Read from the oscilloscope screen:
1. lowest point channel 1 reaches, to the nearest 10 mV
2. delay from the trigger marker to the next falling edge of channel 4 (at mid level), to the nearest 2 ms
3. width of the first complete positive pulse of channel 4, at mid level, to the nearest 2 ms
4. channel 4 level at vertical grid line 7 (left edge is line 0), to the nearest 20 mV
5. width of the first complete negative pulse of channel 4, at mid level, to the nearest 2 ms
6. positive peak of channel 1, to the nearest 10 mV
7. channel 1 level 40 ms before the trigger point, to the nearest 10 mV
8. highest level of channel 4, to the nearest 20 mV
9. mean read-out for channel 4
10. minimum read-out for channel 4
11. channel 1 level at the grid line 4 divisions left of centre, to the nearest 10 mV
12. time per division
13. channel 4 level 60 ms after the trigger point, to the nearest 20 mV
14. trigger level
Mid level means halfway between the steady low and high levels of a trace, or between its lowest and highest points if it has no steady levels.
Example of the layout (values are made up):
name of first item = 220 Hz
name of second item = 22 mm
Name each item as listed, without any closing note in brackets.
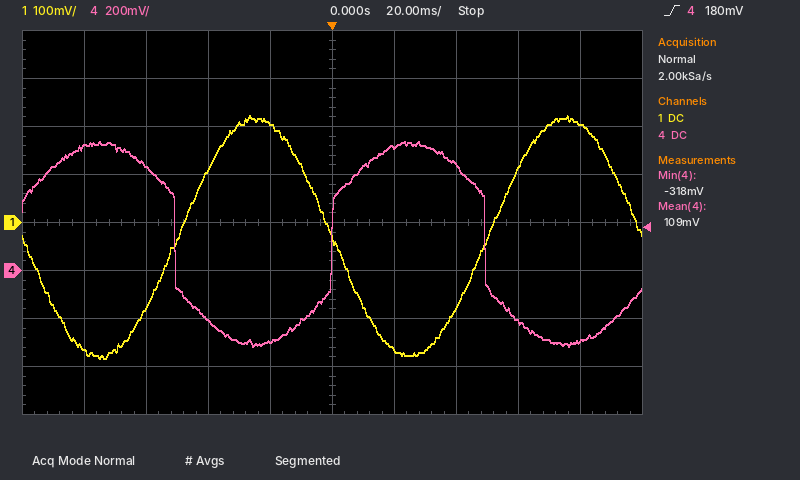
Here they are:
lowest point channel 1 reaches, to the nearest 10 mV = -280 mV
delay from the trigger marker to the next falling edge of channel 4 (at mid level), to the nearest 2 ms = 50 ms
width of the first complete positive pulse of channel 4, at mid level, to the nearest 2 ms = 50 ms
channel 4 level at vertical grid line 7 (left edge is line 0), to the nearest 20 mV = 440 mV
width of the first complete negative pulse of channel 4, at mid level, to the nearest 2 ms = 50 ms
positive peak of channel 1, to the nearest 10 mV = 220 mV
channel 1 level 40 ms before the trigger point, to the nearest 10 mV = 110 mV
highest level of channel 4, to the nearest 20 mV = 540 mV
mean read-out for channel 4 = 109 mV
minimum read-out for channel 4 = -318 mV
channel 1 level at the grid line 4 divisions left of centre, to the nearest 10 mV = -270 mV
time per division = 20 ms
channel 4 level 60 ms after the trigger point, to the nearest 20 mV = -220 mV
trigger level = 180 mV
